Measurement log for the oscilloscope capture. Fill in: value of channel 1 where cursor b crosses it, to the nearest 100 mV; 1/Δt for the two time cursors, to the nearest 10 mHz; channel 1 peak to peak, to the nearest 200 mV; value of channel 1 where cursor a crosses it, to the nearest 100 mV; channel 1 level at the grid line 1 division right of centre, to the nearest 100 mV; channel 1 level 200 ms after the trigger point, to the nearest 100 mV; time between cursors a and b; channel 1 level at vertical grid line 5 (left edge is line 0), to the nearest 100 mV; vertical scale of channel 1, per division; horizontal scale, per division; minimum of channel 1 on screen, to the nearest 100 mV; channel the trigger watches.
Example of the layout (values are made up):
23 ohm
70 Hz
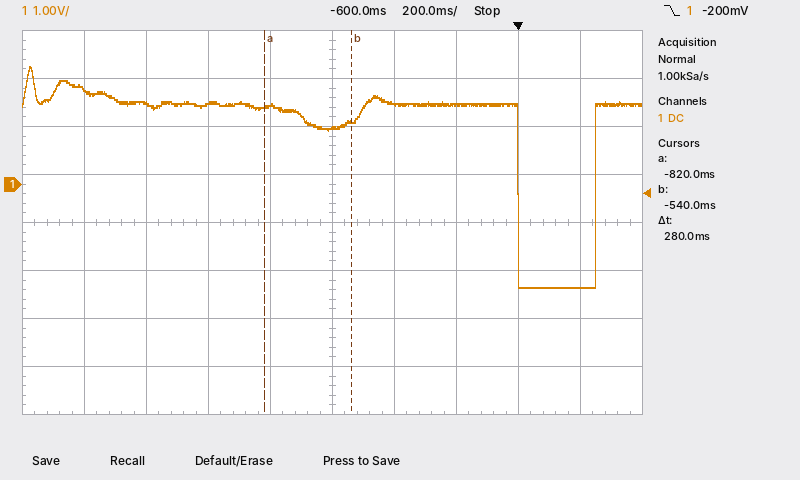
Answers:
1.3 V
3.57 Hz
4.6 V
1.6 V
1.7 V
-2.2 V
280 ms
1.2 V
1 V
200 ms
-2.2 V
channel 1
